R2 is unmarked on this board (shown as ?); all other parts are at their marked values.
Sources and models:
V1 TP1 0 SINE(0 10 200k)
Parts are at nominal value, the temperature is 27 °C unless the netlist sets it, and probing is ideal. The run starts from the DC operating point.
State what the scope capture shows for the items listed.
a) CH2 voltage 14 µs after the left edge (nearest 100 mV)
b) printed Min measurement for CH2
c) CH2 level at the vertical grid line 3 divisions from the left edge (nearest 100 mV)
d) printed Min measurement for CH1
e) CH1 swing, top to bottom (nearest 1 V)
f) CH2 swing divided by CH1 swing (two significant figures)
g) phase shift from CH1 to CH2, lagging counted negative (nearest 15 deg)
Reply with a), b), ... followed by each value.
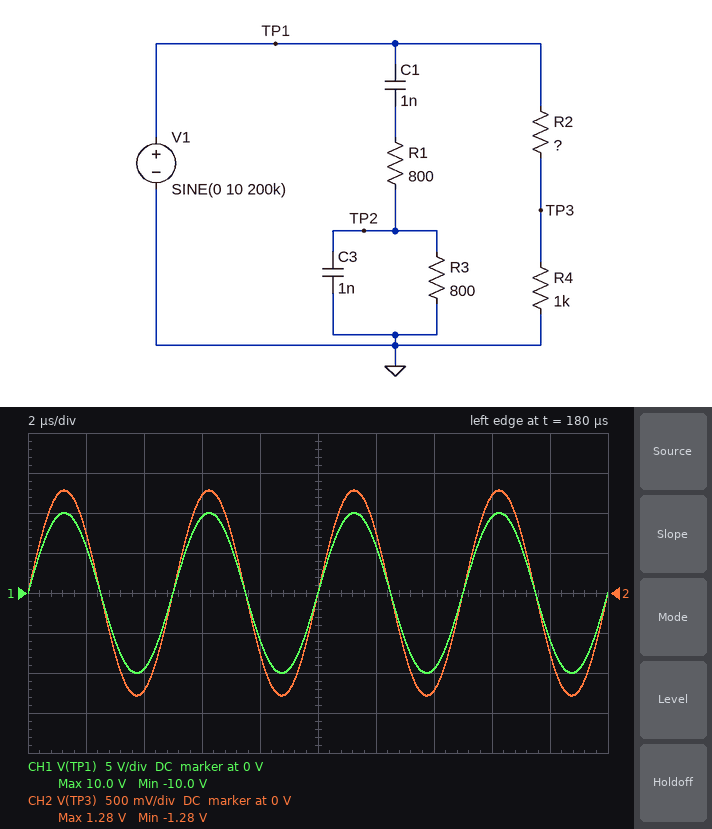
a) -1.2 V
b) -1.28 V
c) 1.2 V
d) -10.0 V
e) 20 V
f) 0.13
g) 0 deg
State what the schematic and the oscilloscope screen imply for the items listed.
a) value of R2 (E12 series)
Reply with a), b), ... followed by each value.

a) 6.8 kΩ
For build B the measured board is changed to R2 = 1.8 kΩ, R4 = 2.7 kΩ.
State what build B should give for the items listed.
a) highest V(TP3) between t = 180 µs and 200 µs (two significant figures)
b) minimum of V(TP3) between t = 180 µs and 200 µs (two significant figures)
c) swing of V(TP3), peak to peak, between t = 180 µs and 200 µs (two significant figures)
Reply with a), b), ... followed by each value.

a) 6.0 V
b) -6.0 V
c) 12 V
